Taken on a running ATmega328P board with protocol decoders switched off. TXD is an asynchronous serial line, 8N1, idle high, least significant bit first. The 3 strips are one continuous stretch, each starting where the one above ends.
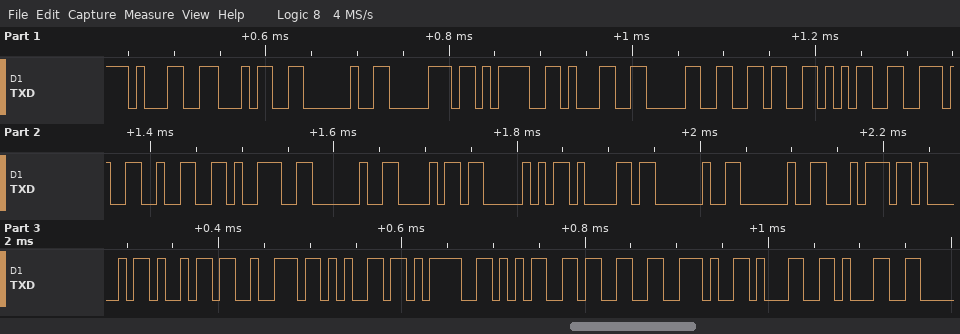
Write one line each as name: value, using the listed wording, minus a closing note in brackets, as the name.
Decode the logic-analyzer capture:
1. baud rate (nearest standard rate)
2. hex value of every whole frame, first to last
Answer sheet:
baud rate: 115200 baud
hex value of every whole frame, first to last: 31 34 20 70 3D 31 30 36 35 2E 32 39 20 68 50 61 20 20 74 41 69 72 65 3D 35 33 2E 31 31
